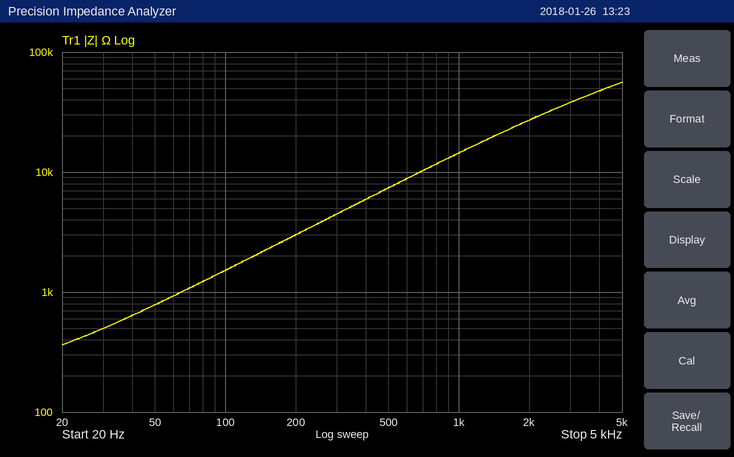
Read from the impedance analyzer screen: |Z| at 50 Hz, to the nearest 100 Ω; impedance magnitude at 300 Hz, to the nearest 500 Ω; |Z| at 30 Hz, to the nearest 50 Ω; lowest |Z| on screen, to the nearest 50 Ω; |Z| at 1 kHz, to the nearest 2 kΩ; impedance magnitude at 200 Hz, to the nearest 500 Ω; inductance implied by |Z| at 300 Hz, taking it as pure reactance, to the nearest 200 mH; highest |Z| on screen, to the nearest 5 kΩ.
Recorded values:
800 Ω
4.5 kΩ
500 Ω
350 Ω
14 kΩ
3.0 kΩ
2.4 H
55 kΩ
